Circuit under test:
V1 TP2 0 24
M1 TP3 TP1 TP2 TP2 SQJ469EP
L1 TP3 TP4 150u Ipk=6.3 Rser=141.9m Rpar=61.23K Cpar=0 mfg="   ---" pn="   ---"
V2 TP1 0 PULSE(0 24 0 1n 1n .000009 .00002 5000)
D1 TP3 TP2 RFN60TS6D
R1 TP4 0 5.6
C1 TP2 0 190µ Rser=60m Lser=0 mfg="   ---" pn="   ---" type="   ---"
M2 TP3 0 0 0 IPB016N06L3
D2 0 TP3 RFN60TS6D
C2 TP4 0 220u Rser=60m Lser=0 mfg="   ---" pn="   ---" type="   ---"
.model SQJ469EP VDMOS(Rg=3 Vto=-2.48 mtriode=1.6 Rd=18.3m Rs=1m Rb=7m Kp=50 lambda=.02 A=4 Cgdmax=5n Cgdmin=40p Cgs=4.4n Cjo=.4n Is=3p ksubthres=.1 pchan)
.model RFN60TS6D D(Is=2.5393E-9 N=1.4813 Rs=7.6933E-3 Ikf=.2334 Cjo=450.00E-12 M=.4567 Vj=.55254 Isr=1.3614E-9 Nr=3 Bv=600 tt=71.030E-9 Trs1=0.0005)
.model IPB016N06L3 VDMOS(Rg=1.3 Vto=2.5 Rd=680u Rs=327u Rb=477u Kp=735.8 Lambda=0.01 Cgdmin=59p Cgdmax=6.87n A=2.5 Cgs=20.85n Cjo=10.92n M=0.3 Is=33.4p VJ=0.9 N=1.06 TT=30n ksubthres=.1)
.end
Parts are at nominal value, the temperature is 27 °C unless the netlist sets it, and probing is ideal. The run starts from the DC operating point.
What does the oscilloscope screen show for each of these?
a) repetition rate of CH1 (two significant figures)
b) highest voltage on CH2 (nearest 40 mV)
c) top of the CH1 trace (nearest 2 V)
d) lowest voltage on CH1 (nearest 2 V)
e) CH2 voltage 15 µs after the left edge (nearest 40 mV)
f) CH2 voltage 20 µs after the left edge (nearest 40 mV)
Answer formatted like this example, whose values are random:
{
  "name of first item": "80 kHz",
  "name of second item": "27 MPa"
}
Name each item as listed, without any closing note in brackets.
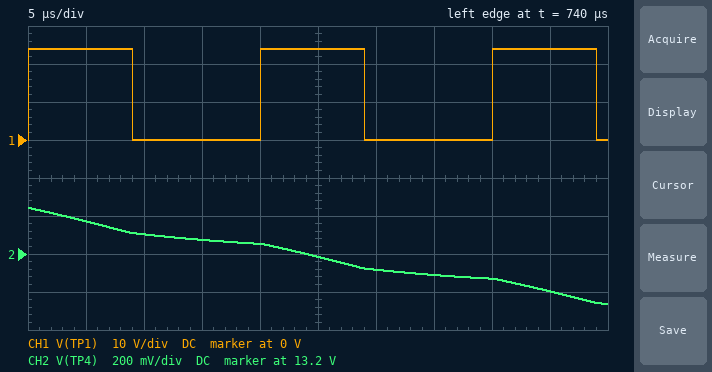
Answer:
{
  "repetition rate of CH1": "50 kHz",
  "highest voltage on CH2": "13.44 V",
  "top of the CH1 trace": "24 V",
  "lowest voltage on CH1": "0 V",
  "CH2 voltage 15 µs after the left edge": "13.28 V",
  "CH2 voltage 20 µs after the left edge": "13.24 V"
}
